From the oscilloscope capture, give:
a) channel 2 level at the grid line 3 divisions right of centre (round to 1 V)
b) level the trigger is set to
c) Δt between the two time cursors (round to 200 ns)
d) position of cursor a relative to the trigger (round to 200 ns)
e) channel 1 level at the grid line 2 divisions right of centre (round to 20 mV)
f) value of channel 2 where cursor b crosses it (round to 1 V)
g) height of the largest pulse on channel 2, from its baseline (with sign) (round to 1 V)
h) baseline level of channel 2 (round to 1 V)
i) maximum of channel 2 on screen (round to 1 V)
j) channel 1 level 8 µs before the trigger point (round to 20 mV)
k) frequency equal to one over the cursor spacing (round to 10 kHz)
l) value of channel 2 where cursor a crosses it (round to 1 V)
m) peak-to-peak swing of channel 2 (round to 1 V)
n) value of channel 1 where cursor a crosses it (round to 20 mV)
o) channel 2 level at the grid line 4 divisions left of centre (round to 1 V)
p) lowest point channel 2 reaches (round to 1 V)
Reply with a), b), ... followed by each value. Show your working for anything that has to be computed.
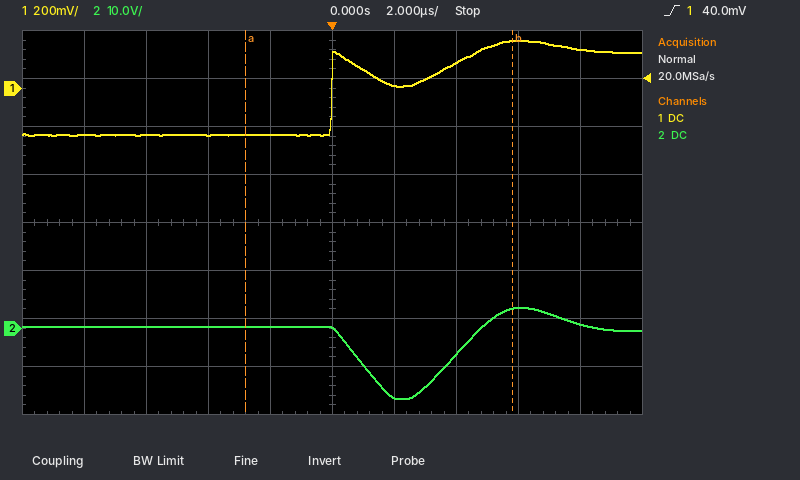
a) 4 V
b) 40.0 mV
c) 8.6 µs
d) -2.8 µs
e) 100 mV
f) 4 V
g) -15 V − (0 V) = -15 V
h) 0 V
i) 4 V
j) -200 mV
k) 1 / 8.6 µs ≈ 120 kHz
l) 0 V
m) 4 V − (-15 V) = 19 V
n) -200 mV
o) 0 V
p) -15 V
